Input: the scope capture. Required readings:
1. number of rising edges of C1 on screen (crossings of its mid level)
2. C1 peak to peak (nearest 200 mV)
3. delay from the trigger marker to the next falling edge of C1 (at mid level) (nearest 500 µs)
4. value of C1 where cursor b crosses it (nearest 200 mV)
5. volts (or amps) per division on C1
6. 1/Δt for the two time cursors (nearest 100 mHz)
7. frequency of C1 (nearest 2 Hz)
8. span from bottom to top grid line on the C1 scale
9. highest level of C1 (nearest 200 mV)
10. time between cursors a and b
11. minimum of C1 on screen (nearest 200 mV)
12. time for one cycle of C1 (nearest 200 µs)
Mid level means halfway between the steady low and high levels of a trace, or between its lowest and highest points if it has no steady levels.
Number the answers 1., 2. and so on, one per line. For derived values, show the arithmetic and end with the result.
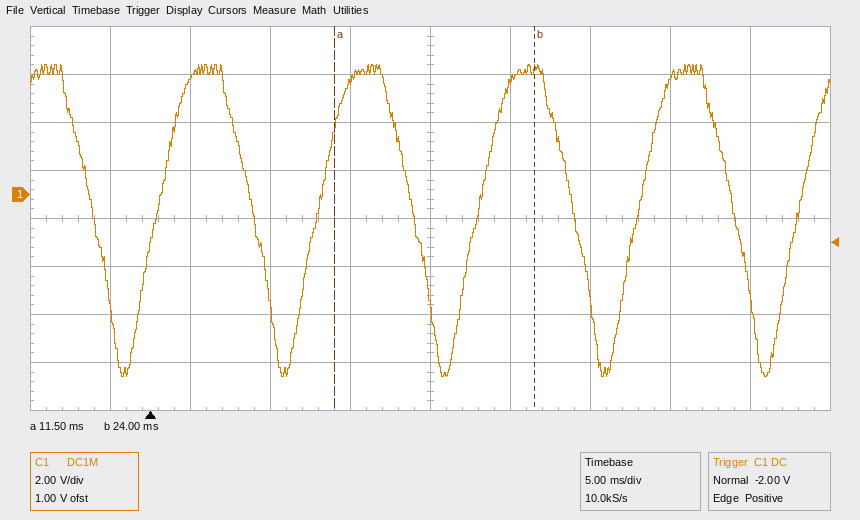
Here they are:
1. 5
2. 5.4 V − (-7.6 V) = 13.0 V
3. 6.5 ms
4. 5.2 V
5. 2 V
6. 1 / 12.5 ms ≈ 80.0 Hz
7. 1 / 10.0 ms ≈ 100 Hz
8. 16 V
9. 5.4 V
10. 24 ms − (11.5 ms) = 12.5 ms
11. -7.6 V
12. 10.0 ms
